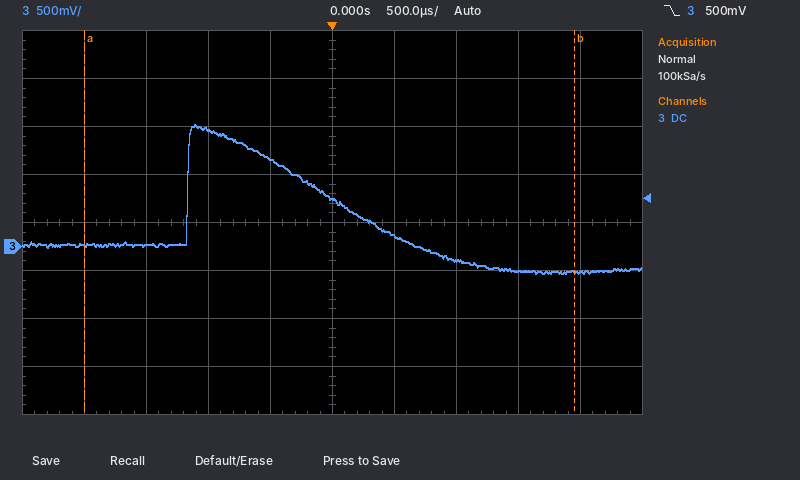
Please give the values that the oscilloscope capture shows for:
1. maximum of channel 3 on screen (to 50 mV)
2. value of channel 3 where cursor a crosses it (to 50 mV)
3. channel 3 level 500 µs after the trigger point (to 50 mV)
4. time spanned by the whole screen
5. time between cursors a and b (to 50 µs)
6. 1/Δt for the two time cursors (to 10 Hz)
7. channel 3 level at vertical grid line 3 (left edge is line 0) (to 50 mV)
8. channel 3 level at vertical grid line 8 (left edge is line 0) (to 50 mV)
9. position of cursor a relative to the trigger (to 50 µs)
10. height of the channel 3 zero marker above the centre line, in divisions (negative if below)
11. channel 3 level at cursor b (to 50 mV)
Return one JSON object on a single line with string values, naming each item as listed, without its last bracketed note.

{"maximum of channel 3 on screen": "1.25 V", "value of channel 3 where cursor a crosses it": "0 mV", "channel 3 level 500 µs after the trigger point": "100 mV", "time spanned by the whole screen": "5 ms", "time between cursors a and b": "3.95 ms", "1/Δt for the two time cursors": "250 Hz", "channel 3 level at vertical grid line 3 (left edge is line 0)": "1.20 V", "channel 3 level at vertical grid line 8 (left edge is line 0)": "-250 mV", "position of cursor a relative to the trigger": "-2.00 ms", "height of the channel 3 zero marker above the centre line, in divisions": "-0.5 div", "channel 3 level at cursor b": "-250 mV"}
